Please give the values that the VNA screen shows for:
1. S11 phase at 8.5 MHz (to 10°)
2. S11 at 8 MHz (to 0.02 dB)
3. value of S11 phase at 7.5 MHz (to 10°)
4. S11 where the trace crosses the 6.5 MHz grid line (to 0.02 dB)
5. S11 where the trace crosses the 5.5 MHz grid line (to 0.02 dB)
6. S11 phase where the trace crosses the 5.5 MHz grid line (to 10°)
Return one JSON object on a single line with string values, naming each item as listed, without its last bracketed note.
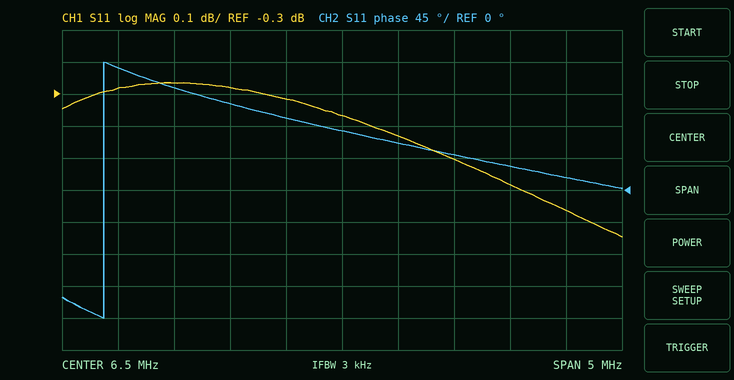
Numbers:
{"S11 phase at 8.5 MHz": "20°", "S11 at 8 MHz": "-0.58 dB", "value of S11 phase at 7.5 MHz": "50°", "S11 where the trace crosses the 6.5 MHz grid line": "-0.36 dB", "S11 where the trace crosses the 5.5 MHz grid line": "-0.28 dB", "S11 phase where the trace crosses the 5.5 MHz grid line": "120°"}
